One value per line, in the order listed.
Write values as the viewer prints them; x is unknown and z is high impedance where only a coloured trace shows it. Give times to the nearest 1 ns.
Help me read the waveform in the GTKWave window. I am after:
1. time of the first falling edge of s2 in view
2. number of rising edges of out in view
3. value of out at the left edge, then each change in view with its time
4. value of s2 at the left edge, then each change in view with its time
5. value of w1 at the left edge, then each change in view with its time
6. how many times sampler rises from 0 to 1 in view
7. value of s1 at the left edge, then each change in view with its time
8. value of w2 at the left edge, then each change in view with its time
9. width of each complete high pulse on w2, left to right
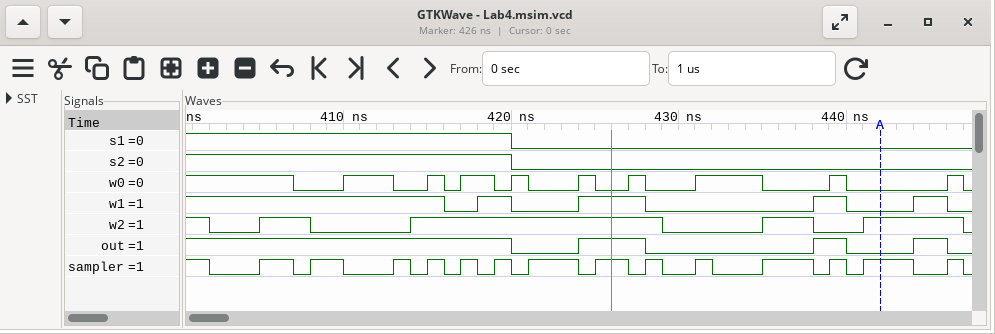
420 ns
3
1, 0 at 420 ns, 1 at 424 ns, 0 at 428 ns, 1 at 438 ns, 0 at 440 ns, 1 at 444 ns, 0 at 446 ns
1, 0 at 420 ns
1, 0 at 416 ns, 1 at 418 ns, 0 at 420 ns, 1 at 424 ns, 0 at 428 ns, 1 at 438 ns, 0 at 440 ns, 1 at 444 ns, 0 at 446 ns
14
1, 0 at 420 ns
1, 0 at 402 ns, 1 at 405 ns, 0 at 408 ns, 1 at 414 ns, 0 at 429 ns, 1 at 435 ns, 0 at 438 ns, 1 at 441 ns, 0 at 447 ns
3 ns, 15 ns, 3 ns, 6 ns
